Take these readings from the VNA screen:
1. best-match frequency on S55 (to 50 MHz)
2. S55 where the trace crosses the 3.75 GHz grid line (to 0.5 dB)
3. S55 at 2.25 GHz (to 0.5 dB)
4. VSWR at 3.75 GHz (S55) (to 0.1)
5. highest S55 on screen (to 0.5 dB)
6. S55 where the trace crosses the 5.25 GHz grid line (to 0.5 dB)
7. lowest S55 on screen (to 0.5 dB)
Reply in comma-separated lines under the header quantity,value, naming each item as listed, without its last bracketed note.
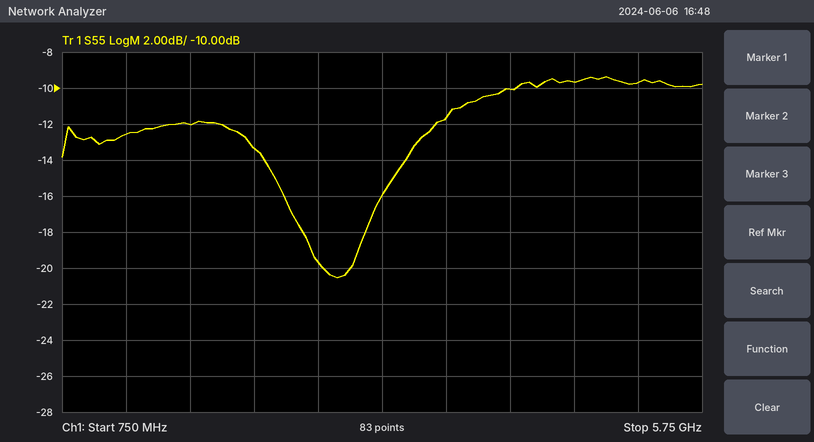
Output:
quantity,value
best-match frequency on S55,2.90 GHz
S55 where the trace crosses the 3.75 GHz grid line,-11.5 dB
S55 at 2.25 GHz,-13.5 dB
VSWR at 3.75 GHz (S55),1.7
highest S55 on screen,-9.5 dB
S55 where the trace crosses the 5.25 GHz grid line,-9.5 dB
lowest S55 on screen,-20.5 dB
